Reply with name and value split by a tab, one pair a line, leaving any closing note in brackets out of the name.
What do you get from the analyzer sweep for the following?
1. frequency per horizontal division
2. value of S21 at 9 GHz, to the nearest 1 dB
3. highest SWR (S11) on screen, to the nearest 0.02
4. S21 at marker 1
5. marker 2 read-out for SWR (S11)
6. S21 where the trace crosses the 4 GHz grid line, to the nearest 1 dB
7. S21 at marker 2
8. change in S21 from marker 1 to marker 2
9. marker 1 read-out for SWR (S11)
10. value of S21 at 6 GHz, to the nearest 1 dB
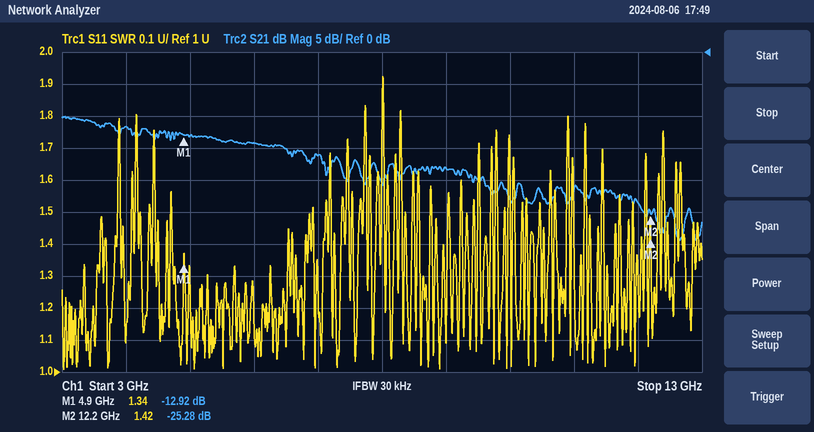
frequency per horizontal division	1 GHz
value of S21 at 9 GHz, to the nearest 1 dB	-18 dB
highest SWR (S11) on screen, to the nearest 0.02	1.92
S21 at marker 1	-12.92 dB
marker 2 read-out for SWR	1.42
S21 where the trace crosses the 4 GHz grid line, to the nearest 1 dB	-12 dB
S21 at marker 2	-25.28 dB
change in S21 from marker 1 to marker 2	-12.36 dB
marker 1 read-out for SWR	1.34
value of S21 at 6 GHz, to the nearest 1 dB	-14 dB
